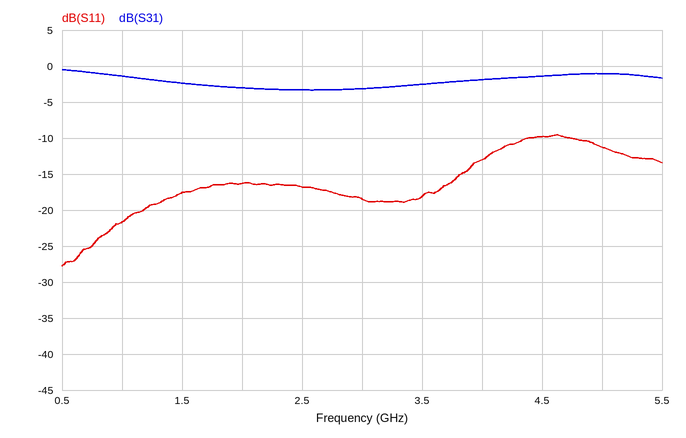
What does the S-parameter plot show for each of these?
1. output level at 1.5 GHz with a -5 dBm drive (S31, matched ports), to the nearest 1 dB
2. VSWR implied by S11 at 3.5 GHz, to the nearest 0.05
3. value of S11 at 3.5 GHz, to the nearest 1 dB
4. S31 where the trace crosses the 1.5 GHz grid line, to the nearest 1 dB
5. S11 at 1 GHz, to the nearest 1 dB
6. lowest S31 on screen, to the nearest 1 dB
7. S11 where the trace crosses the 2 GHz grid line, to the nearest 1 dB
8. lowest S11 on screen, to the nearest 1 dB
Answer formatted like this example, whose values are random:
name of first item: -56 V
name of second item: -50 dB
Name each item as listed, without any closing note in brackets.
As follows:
output level at 1.5 GHz with a -5 dBm drive (S31, matched ports), to the nearest 1 dB: -7 dBm
VSWR implied by S11 at 3.5 GHz, to the nearest 0.05: 1.30
value of S11 at 3.5 GHz, to the nearest 1 dB: -18 dB
S31 where the trace crosses the 1.5 GHz grid line, to the nearest 1 dB: -2 dB
S11 at 1 GHz, to the nearest 1 dB: -22 dB
lowest S31 on screen, to the nearest 1 dB: -3 dB
S11 where the trace crosses the 2 GHz grid line, to the nearest 1 dB: -16 dB
lowest S11 on screen, to the nearest 1 dB: -28 dB
